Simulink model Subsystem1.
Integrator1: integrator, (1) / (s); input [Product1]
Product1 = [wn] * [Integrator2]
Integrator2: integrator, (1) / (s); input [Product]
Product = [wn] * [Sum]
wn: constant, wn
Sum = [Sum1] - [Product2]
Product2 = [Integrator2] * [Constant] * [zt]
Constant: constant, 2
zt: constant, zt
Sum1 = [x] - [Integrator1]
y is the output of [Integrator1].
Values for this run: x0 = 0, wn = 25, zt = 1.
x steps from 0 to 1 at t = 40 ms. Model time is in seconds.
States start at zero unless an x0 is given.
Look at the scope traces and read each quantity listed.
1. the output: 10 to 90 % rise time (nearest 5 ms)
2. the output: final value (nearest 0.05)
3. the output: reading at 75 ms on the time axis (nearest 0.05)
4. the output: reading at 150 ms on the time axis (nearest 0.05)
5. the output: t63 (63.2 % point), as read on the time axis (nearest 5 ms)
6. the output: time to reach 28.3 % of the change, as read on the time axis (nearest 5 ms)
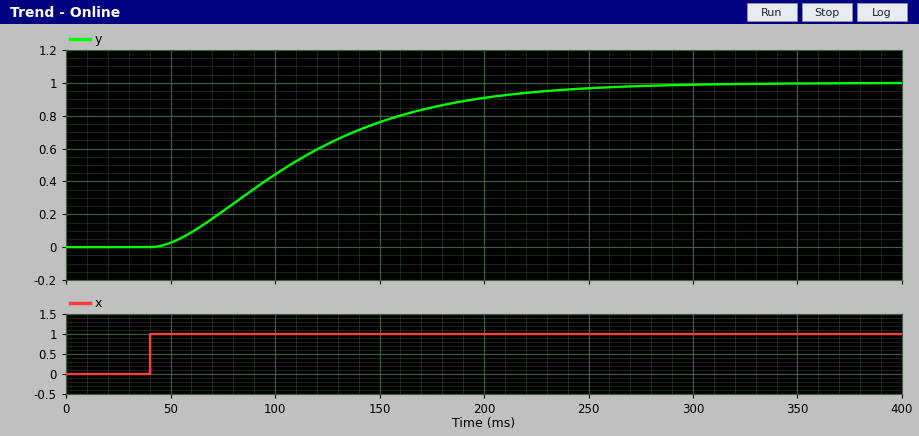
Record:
135 ms
1.00
0.20
0.75
125 ms
80 ms
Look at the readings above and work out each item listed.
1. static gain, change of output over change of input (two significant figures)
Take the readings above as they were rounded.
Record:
1.0
